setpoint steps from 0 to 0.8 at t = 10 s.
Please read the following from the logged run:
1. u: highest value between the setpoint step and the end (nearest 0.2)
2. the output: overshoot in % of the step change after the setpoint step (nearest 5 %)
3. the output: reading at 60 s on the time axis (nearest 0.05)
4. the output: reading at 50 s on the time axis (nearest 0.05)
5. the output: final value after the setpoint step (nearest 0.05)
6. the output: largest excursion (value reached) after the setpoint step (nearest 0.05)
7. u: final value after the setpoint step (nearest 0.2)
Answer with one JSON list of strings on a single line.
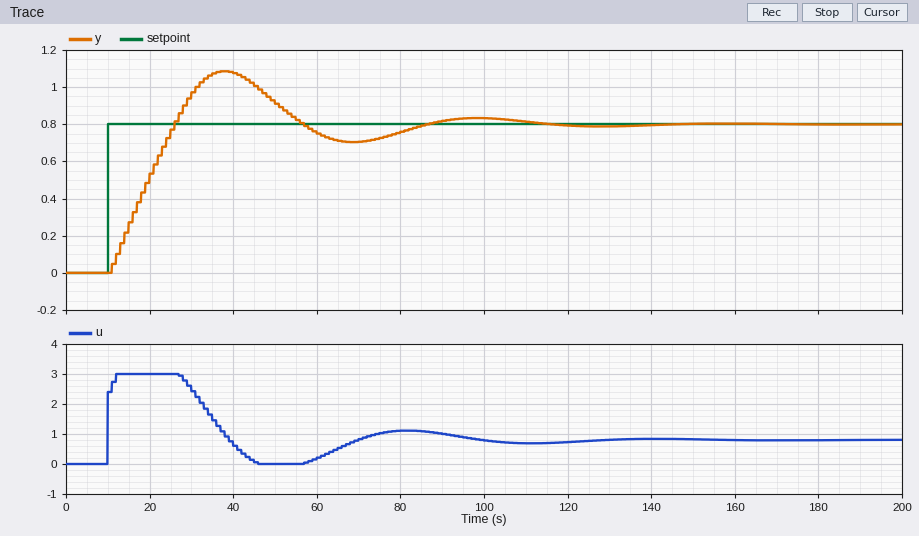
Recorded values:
["3.0", "35 %", "0.75", "0.90", "0.80", "1.10", "0.8"]
